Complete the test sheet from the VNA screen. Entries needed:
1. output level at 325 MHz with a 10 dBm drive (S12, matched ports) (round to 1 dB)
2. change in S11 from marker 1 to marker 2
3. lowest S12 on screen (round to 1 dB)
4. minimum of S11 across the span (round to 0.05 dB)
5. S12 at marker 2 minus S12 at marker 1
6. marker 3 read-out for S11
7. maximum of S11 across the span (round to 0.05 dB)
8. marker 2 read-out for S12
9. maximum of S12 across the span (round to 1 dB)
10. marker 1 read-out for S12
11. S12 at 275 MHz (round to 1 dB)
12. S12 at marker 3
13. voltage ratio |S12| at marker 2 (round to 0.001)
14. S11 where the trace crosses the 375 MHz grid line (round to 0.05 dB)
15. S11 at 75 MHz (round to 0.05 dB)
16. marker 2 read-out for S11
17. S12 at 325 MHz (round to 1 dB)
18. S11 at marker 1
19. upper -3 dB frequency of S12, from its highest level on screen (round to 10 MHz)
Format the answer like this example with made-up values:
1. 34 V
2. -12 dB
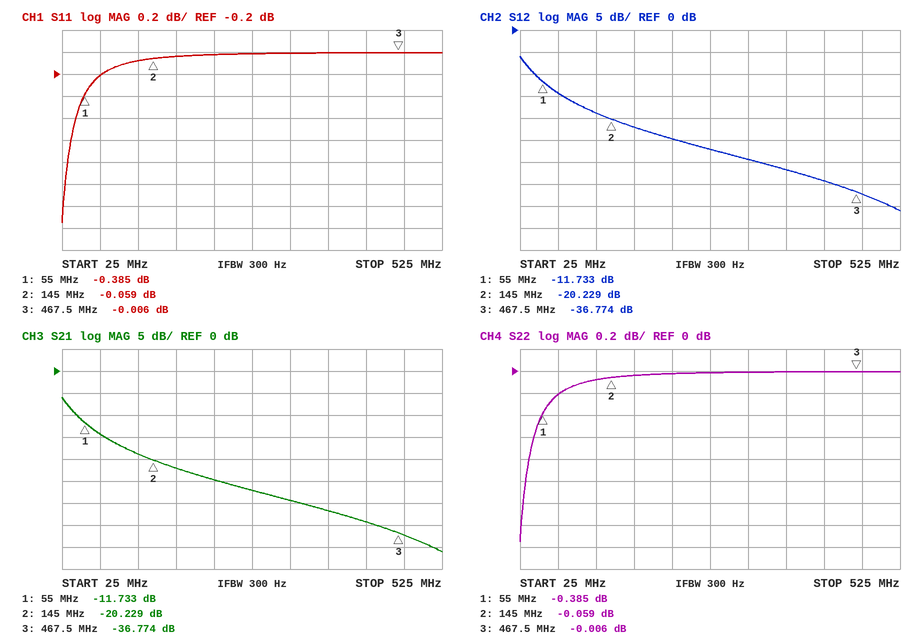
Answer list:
1. -19 dBm
2. 0.326 dB
3. -41 dB
4. -1.55 dB
5. -8.496 dB
6. -0.006 dB
7. 0.00 dB
8. -20.229 dB
9. -6 dB
10. -11.733 dB
11. -27 dB
12. -36.774 dB
13. 0.097
14. 0.00 dB
15. -0.20 dB
16. -0.059 dB
17. -29 dB
18. -0.385 dB
19. 40 MHz
